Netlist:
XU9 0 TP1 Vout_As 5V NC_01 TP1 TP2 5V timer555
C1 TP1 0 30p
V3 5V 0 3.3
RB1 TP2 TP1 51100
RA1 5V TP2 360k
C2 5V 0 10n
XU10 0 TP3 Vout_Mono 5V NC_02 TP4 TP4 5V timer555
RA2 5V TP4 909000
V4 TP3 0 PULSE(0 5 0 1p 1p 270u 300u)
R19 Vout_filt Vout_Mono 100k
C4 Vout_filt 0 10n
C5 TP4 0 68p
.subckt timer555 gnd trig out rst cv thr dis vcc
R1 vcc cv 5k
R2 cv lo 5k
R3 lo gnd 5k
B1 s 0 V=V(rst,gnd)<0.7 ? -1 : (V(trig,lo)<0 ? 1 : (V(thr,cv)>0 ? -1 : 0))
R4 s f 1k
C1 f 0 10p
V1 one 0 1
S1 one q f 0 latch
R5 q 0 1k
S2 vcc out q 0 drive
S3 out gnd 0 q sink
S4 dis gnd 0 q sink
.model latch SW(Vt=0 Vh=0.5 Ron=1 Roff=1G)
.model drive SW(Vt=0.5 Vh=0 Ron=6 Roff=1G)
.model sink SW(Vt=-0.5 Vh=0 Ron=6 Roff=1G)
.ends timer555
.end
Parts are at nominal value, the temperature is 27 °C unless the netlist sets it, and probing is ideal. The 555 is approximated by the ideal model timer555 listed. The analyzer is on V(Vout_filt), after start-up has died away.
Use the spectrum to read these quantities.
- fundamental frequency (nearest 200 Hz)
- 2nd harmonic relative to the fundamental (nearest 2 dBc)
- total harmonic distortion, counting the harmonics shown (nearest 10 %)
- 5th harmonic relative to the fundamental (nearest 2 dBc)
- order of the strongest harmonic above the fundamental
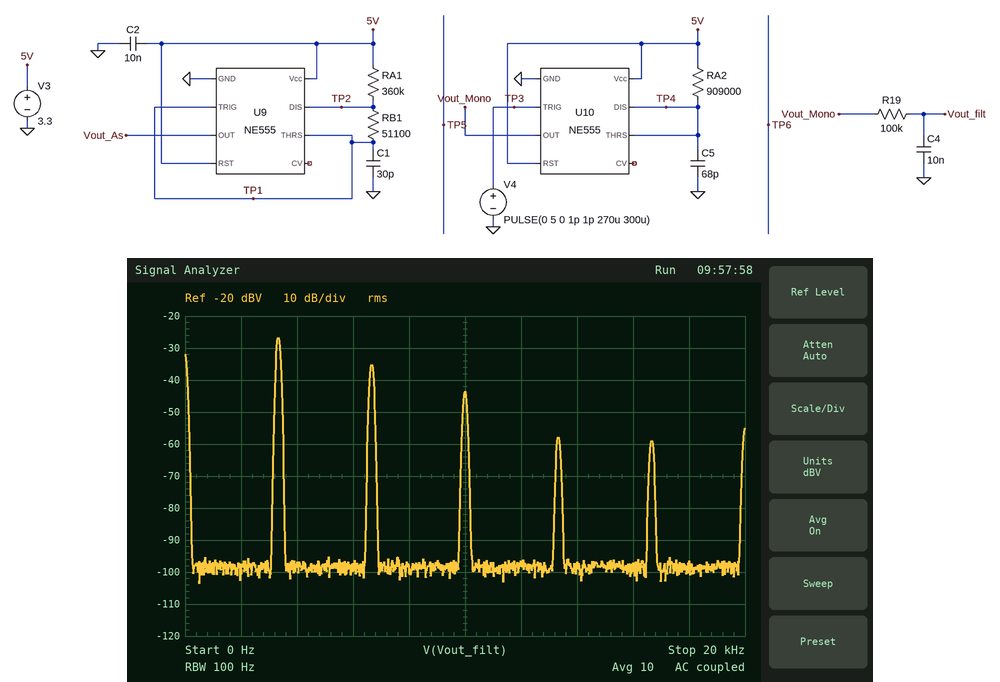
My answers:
3.4 kHz
-8 dBc
40 %
-32 dBc
2
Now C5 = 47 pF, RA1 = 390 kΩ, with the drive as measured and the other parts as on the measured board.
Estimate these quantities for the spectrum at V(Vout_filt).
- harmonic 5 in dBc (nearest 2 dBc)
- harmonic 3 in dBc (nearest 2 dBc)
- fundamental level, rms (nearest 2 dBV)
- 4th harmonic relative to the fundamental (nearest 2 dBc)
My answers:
-26 dBc
-12 dBc
-30 dBV
-18 dBc
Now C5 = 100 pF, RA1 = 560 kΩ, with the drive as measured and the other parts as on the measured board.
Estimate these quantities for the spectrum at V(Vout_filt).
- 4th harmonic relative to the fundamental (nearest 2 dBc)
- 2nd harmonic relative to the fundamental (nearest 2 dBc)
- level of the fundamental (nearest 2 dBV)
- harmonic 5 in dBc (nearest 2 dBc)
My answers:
-24 dBc
-12 dBc
-24 dBV
-28 dBc
